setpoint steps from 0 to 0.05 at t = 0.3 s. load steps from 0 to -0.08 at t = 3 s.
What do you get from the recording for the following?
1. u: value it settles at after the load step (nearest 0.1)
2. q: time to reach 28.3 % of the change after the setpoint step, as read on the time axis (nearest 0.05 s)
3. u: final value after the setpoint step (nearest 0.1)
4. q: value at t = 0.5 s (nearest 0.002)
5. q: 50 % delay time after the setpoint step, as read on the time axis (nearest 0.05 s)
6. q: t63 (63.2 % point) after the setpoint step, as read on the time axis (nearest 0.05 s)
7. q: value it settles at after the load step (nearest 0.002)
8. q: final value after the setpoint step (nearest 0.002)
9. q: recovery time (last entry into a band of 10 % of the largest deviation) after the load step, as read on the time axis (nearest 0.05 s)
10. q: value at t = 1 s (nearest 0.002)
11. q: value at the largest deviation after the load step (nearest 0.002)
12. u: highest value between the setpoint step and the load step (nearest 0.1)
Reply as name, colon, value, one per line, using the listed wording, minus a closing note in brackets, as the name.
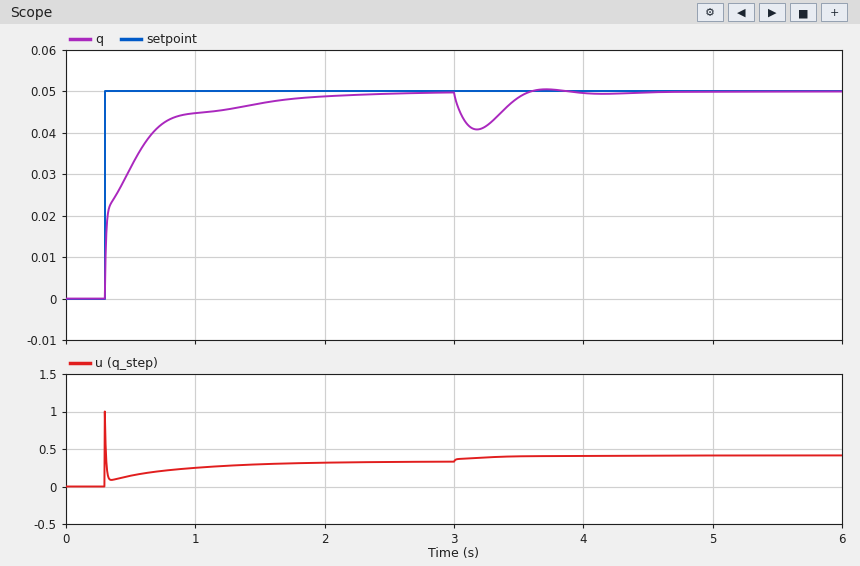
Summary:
u: value it settles at after the load step: 0.4
q: time to reach 28.3 % of the change after the setpoint step, as read on the time axis: 0.30 s
u: final value after the setpoint step: 0.3
q: value at t = 0.5 s: 0.032
q: 50 % delay time after the setpoint step, as read on the time axis: 0.40 s
q: t63 (63.2 % point) after the setpoint step, as read on the time axis: 0.50 s
q: value it settles at after the load step: 0.050
q: final value after the setpoint step: 0.050
q: recovery time (last entry into a band of 10 % of the largest deviation) after the load step, as read on the time axis: 3.55 s
q: value at t = 1 s: 0.044
q: value at the largest deviation after the load step: 0.040
u: highest value between the setpoint step and the load step: 1.0
